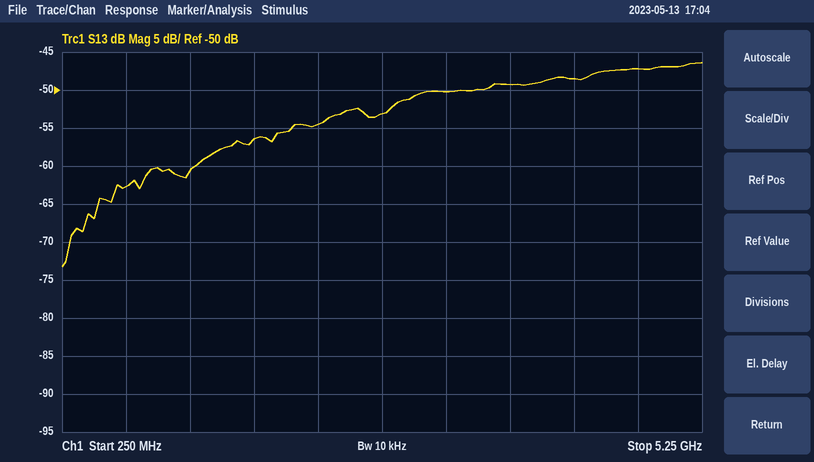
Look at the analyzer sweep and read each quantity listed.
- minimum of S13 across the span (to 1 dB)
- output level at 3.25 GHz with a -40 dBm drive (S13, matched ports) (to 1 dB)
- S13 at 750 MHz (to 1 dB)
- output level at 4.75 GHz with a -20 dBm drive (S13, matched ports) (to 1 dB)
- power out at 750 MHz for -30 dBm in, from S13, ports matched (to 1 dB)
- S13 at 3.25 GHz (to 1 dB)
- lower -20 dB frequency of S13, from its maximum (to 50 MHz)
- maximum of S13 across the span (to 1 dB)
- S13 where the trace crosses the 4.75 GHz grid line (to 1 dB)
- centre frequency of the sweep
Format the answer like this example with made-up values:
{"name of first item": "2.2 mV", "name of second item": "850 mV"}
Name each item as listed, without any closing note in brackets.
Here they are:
{"minimum of S13 across the span": "-73 dB", "output level at 3.25 GHz with a -40 dBm drive (S13, matched ports)": "-90 dBm", "S13 at 750 MHz": "-63 dB", "output level at 4.75 GHz with a -20 dBm drive (S13, matched ports)": "-67 dBm", "power out at 750 MHz for -30 dBm in, from S13, ports matched": "-93 dBm", "S13 at 3.25 GHz": "-50 dB", "lower -20 dB frequency of S13, from its maximum": "500 MHz", "maximum of S13 across the span": "-46 dB", "S13 where the trace crosses the 4.75 GHz grid line": "-47 dB", "centre frequency of the sweep": "2.75 GHz"}
